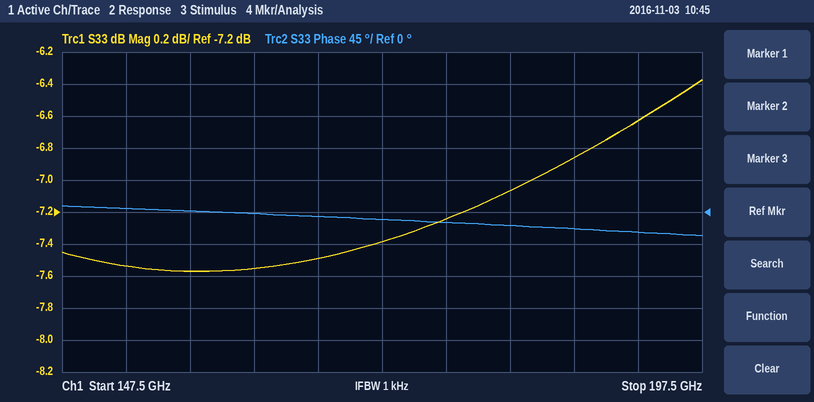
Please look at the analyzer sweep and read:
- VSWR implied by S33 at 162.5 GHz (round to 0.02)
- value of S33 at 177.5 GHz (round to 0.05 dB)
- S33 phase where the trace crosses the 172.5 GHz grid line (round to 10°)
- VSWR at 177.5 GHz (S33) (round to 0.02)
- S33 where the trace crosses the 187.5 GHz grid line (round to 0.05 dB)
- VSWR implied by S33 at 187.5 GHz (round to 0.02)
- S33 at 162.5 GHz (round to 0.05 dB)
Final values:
2.44
-7.25 dB
-10°
2.54
-6.85 dB
2.66
-7.55 dB
